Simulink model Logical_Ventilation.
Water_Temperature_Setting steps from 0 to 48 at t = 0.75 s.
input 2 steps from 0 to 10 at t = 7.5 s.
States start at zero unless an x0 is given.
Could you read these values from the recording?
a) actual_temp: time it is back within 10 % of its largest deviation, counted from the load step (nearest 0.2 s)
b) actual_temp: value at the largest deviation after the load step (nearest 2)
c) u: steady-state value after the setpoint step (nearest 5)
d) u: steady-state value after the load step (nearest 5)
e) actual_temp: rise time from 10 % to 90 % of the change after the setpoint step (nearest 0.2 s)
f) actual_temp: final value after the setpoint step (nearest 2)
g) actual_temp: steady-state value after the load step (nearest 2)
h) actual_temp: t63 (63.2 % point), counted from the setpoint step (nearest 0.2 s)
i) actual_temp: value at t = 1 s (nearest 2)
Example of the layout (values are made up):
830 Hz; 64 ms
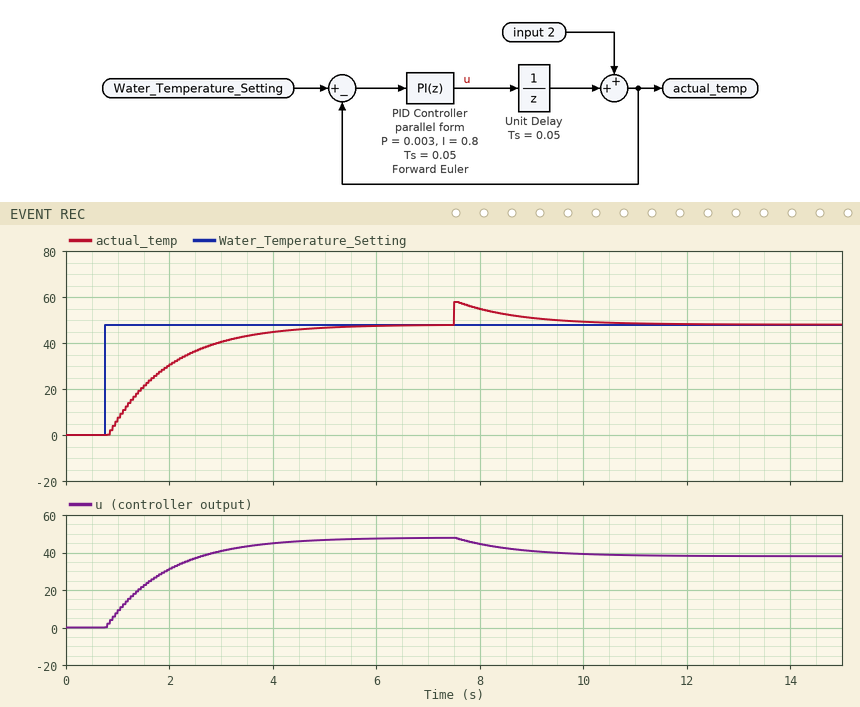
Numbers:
2.8 s; 58; 50; 40; 2.6 s; 48; 48; 1.2 s; 8
